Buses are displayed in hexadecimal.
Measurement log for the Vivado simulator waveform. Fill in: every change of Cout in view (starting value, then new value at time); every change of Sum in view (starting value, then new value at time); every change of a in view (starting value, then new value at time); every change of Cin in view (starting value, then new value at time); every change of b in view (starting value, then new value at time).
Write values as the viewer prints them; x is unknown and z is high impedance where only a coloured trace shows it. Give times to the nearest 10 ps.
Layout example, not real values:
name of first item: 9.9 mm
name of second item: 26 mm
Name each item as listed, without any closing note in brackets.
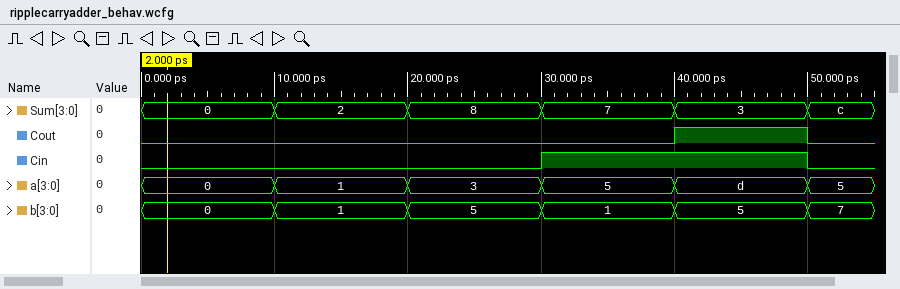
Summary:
every change of Cout in view: 0, 1 at 40 ps, 0 at 50 ps
every change of Sum in view: 0, 2 at 10 ps, 8 at 20 ps, 7 at 30 ps, 3 at 40 ps, c at 50 ps
every change of a in view: 0, 1 at 10 ps, 3 at 20 ps, 5 at 30 ps, d at 40 ps, 5 at 50 ps
every change of Cin in view: 0, 1 at 30 ps, 0 at 50 ps
every change of b in view: 0, 1 at 10 ps, 5 at 20 ps, 1 at 30 ps, 5 at 40 ps, 7 at 50 ps
